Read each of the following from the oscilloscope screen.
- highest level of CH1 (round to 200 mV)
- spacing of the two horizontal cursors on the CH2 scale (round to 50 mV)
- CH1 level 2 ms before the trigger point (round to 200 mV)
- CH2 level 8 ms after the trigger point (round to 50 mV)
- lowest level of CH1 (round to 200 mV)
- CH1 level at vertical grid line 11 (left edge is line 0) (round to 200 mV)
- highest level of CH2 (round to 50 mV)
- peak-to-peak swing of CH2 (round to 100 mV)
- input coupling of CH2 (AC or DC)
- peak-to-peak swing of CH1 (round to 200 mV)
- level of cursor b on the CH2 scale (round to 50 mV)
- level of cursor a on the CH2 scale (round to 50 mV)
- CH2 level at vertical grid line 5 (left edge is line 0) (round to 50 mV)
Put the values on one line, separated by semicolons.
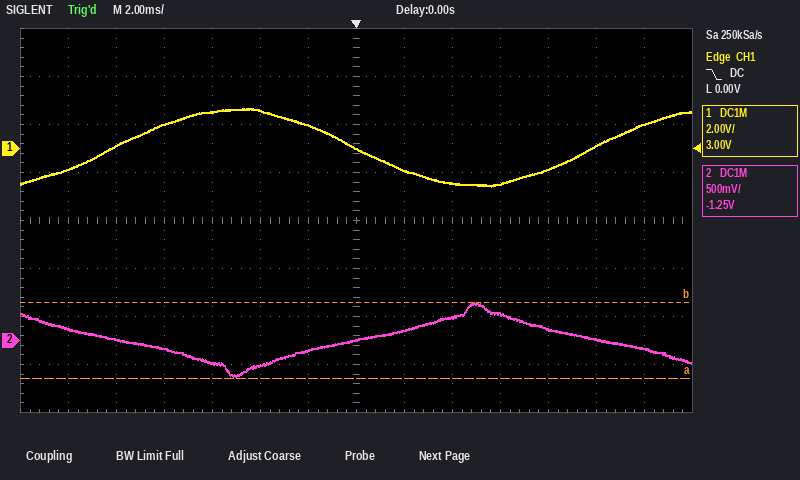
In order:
1.6 V; 800 mV; 1.0 V; 100 mV; -1.6 V; -800 mV; 400 mV; 800 mV; DC; 3.2 V; 400 mV; -400 mV; -250 mV
